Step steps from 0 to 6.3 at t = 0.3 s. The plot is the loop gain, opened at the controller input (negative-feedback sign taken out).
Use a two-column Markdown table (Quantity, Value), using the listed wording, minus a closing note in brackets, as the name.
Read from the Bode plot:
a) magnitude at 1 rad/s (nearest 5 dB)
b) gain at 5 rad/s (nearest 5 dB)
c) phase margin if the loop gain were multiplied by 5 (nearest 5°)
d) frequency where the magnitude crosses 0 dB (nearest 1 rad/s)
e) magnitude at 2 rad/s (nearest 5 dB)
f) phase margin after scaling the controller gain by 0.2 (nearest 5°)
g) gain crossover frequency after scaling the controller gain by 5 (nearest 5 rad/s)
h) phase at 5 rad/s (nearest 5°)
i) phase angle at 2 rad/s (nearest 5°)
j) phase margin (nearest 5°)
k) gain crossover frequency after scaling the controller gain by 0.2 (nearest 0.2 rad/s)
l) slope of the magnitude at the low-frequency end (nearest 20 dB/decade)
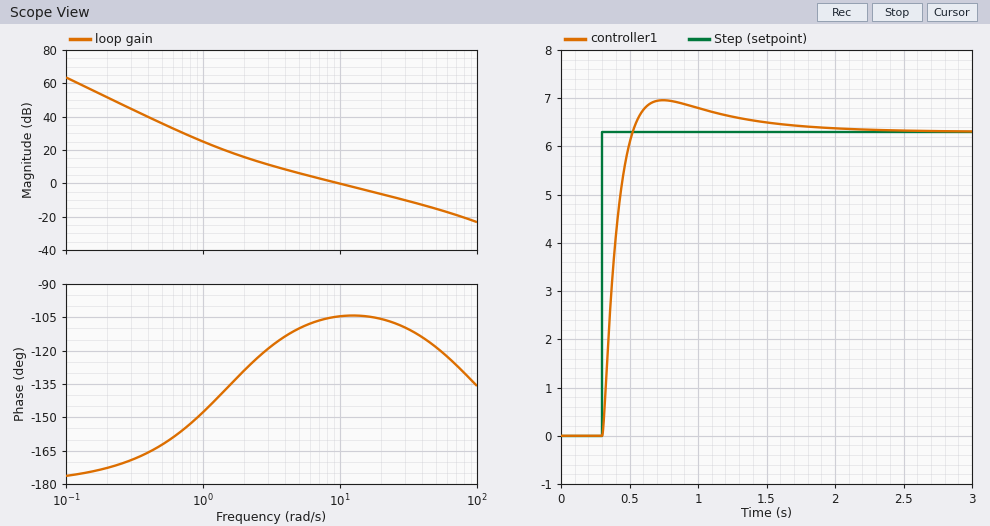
| Quantity | Value |
|---|---|
| magnitude at 1 rad/s | 25 dB |
| gain at 5 rad/s | 5 dB |
| phase margin if the loop gain were multiplied by 5 | 65° |
| frequency where the magnitude crosses 0 dB | 10 rad/s |
| magnitude at 2 rad/s | 15 dB |
| phase margin after scaling the controller gain by 0.2 | 55° |
| gain crossover frequency after scaling the controller gain by 5 | 45 rad/s |
| phase at 5 rad/s | -110° |
| phase angle at 2 rad/s | -130° |
| phase margin | 75° |
| gain crossover frequency after scaling the controller gain by 0.2 | 2.4 rad/s |
| slope of the magnitude at the low-frequency end | -40 dB/decade |
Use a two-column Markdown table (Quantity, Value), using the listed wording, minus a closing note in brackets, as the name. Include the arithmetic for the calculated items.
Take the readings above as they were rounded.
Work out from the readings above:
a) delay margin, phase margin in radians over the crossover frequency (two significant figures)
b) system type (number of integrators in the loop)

| Quantity | Value |
|---|---|
| delay margin, phase margin in radians over the crossover frequency | 75 × π / 180 / 10 = 0.13 s |
| system type | 2 |
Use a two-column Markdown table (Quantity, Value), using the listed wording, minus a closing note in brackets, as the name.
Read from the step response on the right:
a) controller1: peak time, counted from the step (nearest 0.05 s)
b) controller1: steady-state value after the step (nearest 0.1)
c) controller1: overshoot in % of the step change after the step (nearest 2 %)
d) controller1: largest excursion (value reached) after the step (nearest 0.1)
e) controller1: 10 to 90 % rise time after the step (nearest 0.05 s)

| Quantity | Value |
|---|---|
| controller1: peak time, counted from the step | 0.45 s |
| controller1: steady-state value after the step | 6.3 |
| controller1: overshoot in % of the step change after the step | 10 % |
| controller1: largest excursion (value reached) after the step | 7.0 |
| controller1: 10 to 90 % rise time after the step | 0.15 s |
